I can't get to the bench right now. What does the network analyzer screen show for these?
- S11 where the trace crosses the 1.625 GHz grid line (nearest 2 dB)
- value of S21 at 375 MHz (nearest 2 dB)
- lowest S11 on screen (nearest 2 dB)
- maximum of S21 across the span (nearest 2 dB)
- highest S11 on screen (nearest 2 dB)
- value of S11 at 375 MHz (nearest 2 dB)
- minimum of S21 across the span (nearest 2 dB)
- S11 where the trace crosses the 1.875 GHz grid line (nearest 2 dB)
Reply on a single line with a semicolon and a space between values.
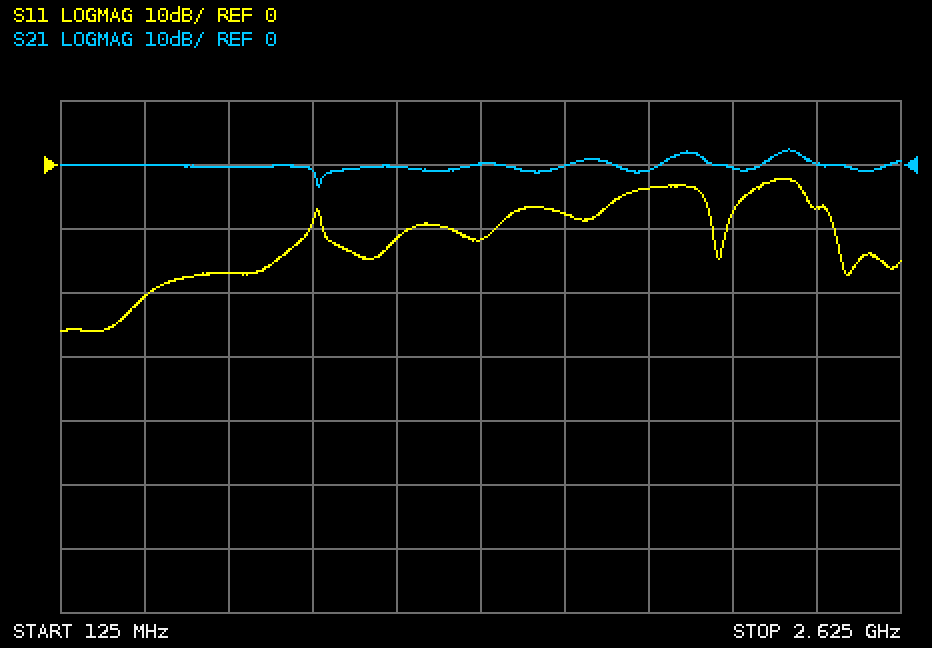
-8 dB; 0 dB; -26 dB; 2 dB; -2 dB; -20 dB; -4 dB; -4 dB
